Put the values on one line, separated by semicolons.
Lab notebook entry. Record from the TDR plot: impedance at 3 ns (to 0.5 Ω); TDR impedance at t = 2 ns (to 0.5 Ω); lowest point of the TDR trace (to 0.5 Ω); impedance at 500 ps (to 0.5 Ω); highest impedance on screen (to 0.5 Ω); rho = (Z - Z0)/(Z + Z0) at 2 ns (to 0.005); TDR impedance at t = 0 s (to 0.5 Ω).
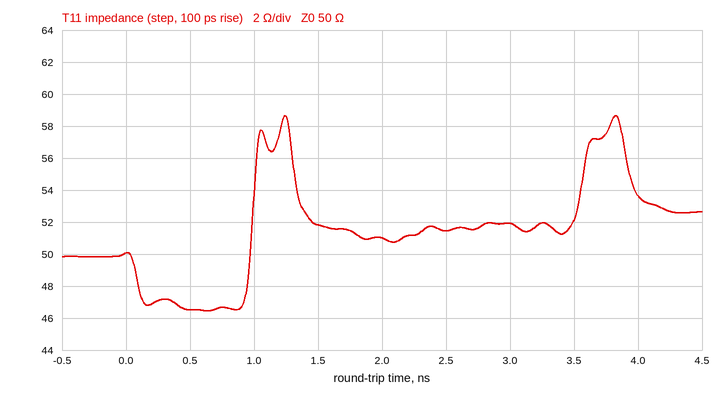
52.0 Ω; 51.0 Ω; 46.5 Ω; 46.5 Ω; 58.5 Ω; +0.010; 50.0 Ω
